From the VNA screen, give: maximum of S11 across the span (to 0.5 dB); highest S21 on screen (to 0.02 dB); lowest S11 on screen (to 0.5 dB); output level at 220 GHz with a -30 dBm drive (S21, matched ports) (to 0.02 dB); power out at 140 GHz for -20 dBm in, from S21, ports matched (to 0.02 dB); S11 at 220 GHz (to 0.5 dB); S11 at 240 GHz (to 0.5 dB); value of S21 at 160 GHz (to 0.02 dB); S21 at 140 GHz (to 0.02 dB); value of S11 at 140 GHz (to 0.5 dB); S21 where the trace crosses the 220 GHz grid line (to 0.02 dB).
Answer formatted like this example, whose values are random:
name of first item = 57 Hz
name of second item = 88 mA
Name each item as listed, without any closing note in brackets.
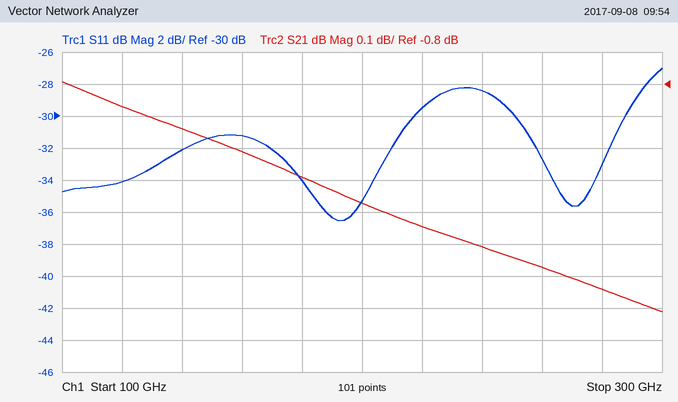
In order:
maximum of S11 across the span = -27.0 dB
highest S21 on screen = -0.80 dB
lowest S11 on screen = -36.5 dB
output level at 220 GHz with a -30 dBm drive (S21, matched ports) = -31.24 dBm
power out at 140 GHz for -20 dBm in, from S21, ports matched = -20.94 dBm
S11 at 220 GHz = -29.5 dB
S11 at 240 GHz = -28.5 dB
value of S21 at 160 GHz = -1.02 dB
S21 at 140 GHz = -0.94 dB
value of S11 at 140 GHz = -32.0 dB
S21 where the trace crosses the 220 GHz grid line = -1.24 dB
